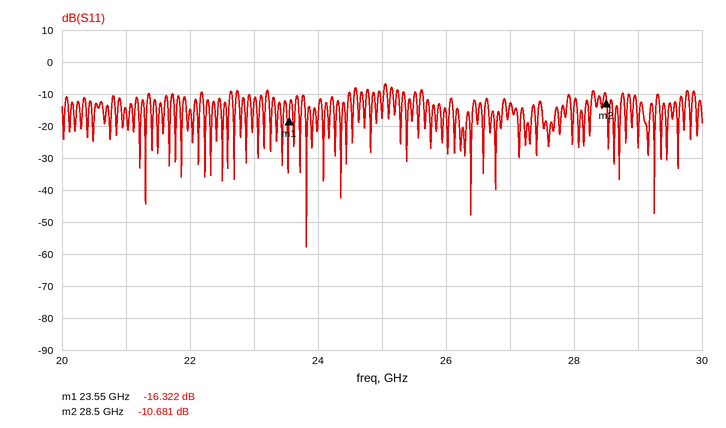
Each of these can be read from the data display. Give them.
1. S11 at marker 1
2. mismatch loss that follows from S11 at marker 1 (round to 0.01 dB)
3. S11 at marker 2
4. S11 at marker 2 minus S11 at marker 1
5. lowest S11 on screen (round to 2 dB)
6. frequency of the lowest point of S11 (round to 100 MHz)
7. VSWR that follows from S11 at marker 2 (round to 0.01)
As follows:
-16.322 dB
0.10 dB
-10.681 dB
5.641 dB
-58 dB
23.8 GHz
1.83
